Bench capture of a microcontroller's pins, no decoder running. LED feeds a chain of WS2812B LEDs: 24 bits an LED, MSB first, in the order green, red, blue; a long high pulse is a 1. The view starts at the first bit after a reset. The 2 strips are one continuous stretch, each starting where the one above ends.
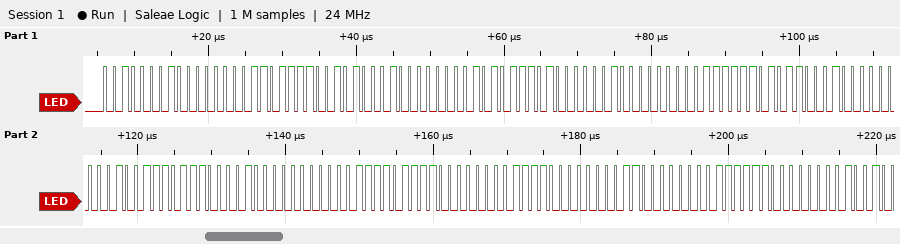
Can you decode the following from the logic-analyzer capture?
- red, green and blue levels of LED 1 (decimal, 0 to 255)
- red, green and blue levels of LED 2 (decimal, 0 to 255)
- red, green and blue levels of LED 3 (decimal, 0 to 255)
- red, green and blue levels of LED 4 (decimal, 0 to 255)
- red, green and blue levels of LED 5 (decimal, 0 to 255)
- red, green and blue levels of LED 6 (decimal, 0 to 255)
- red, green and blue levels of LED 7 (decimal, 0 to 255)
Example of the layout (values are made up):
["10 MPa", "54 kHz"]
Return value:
["0, 33, 222", "0, 81, 174", "0, 129, 126", "0, 177, 78", "0, 225, 30", "15, 240, 0", "63, 192, 0"]
